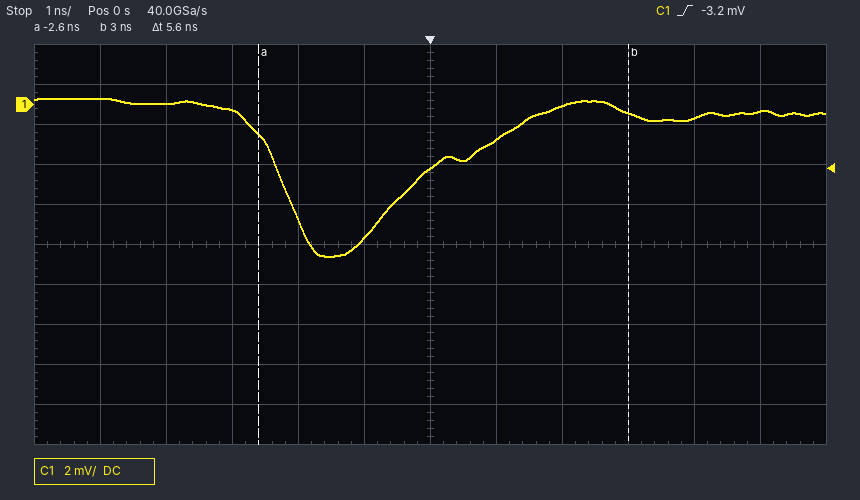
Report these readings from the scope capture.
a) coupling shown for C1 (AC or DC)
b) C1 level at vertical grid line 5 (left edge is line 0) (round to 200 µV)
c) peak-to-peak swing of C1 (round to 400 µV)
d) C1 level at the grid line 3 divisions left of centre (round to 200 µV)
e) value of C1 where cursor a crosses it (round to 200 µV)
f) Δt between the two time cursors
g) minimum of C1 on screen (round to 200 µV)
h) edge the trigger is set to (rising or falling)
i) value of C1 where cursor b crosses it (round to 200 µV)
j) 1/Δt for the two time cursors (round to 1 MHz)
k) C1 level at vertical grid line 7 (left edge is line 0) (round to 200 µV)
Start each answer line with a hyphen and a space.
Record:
- DC
- -6.6 mV
- 8.0 mV
- -200 µV
- -1.4 mV
- 5.6 ns
- -7.6 mV
- rising
- -400 µV
- 179 MHz
- -1.8 mV
